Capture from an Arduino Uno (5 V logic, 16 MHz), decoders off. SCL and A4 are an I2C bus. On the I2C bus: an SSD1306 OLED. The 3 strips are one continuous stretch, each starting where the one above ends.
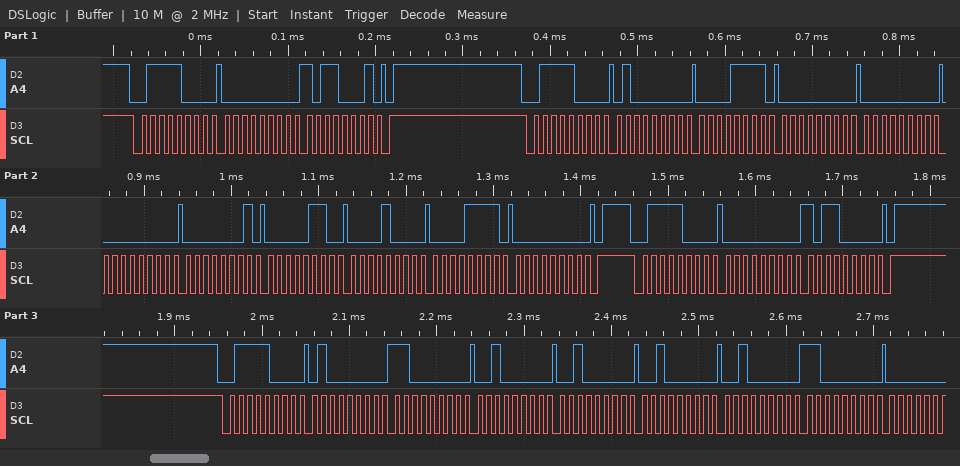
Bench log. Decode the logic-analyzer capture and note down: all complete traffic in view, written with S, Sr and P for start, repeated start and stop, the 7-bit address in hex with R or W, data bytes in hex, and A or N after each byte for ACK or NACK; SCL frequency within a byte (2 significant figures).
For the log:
S 3CW A 00 A B1 A P S 3CW A 40 A 0F A 00 A 00 A 00 A 01 A 06 A 08 A 0F A 00 A P S 3CW A 00 A B0 A P S 3CW A 40 A C0 A 20 A 20 A 20 A 20 A C0 A
100 kHz
